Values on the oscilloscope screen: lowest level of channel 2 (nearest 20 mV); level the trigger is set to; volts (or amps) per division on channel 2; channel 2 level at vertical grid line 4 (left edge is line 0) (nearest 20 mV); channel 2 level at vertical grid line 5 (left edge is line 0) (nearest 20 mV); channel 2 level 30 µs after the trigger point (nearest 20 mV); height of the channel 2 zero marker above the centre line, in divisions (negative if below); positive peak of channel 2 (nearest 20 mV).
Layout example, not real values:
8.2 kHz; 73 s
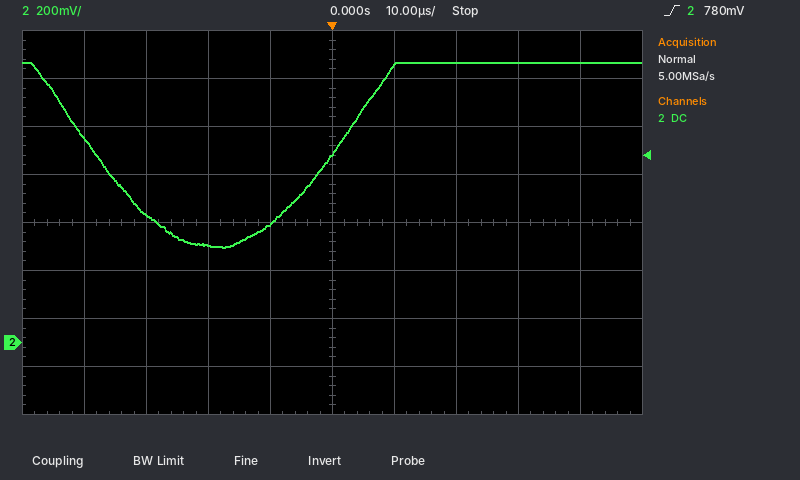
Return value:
400 mV; 780 mV; 200 mV; 500 mV; 780 mV; 1.16 V; -2.5 div; 1.16 V
